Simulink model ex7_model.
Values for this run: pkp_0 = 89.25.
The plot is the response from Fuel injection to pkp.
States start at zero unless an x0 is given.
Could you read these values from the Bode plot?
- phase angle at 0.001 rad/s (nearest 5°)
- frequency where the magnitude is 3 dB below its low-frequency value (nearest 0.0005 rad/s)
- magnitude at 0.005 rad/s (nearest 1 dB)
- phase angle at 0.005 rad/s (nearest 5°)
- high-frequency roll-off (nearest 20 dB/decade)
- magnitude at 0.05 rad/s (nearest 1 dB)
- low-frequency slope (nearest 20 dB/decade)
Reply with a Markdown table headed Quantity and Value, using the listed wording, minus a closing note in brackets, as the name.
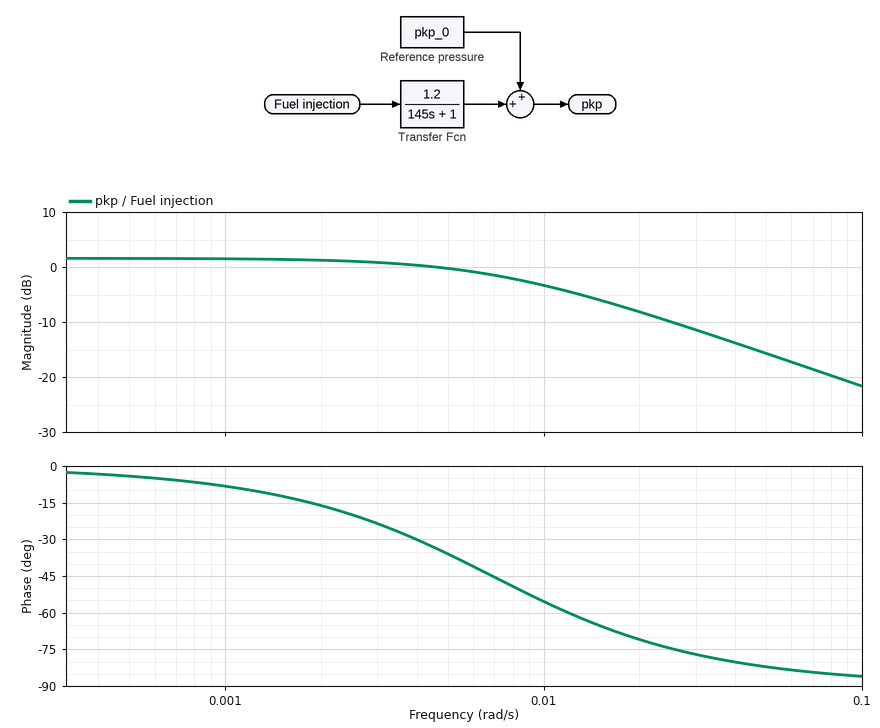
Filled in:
| Quantity | Value |
|---|---|
| phase angle at 0.001 rad/s | -10° |
| frequency where the magnitude is 3 dB below its low-frequency value | 0.0070 rad/s |
| magnitude at 0.005 rad/s | 0 dB |
| phase angle at 0.005 rad/s | -35° |
| high-frequency roll-off | -20 dB/decade |
| magnitude at 0.05 rad/s | -16 dB |
| low-frequency slope | 0 dB/decade |
